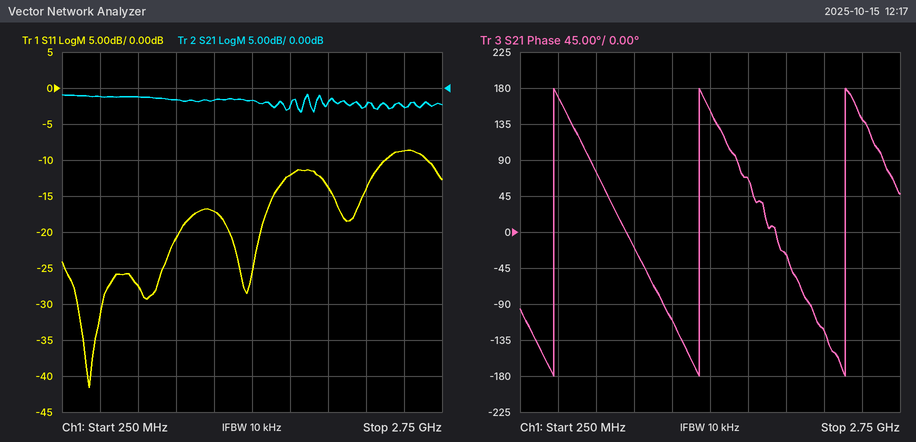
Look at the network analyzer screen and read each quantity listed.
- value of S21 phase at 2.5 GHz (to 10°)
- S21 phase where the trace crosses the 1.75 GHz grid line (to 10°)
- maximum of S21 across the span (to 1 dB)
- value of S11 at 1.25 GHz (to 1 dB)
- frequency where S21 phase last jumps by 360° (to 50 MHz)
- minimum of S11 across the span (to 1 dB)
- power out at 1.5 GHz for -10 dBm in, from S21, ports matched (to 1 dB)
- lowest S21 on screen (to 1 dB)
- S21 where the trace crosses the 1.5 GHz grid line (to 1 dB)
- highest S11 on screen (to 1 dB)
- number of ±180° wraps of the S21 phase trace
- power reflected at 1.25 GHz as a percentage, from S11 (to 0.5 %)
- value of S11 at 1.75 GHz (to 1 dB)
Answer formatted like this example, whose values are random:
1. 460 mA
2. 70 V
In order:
1. 140°
2. 70°
3. -1 dB
4. -17 dB
5. 2.40 GHz
6. -42 dB
7. -12 dBm
8. -3 dB
9. -2 dB
10. -9 dB
11. 3
12. 2.0 %
13. -12 dB
